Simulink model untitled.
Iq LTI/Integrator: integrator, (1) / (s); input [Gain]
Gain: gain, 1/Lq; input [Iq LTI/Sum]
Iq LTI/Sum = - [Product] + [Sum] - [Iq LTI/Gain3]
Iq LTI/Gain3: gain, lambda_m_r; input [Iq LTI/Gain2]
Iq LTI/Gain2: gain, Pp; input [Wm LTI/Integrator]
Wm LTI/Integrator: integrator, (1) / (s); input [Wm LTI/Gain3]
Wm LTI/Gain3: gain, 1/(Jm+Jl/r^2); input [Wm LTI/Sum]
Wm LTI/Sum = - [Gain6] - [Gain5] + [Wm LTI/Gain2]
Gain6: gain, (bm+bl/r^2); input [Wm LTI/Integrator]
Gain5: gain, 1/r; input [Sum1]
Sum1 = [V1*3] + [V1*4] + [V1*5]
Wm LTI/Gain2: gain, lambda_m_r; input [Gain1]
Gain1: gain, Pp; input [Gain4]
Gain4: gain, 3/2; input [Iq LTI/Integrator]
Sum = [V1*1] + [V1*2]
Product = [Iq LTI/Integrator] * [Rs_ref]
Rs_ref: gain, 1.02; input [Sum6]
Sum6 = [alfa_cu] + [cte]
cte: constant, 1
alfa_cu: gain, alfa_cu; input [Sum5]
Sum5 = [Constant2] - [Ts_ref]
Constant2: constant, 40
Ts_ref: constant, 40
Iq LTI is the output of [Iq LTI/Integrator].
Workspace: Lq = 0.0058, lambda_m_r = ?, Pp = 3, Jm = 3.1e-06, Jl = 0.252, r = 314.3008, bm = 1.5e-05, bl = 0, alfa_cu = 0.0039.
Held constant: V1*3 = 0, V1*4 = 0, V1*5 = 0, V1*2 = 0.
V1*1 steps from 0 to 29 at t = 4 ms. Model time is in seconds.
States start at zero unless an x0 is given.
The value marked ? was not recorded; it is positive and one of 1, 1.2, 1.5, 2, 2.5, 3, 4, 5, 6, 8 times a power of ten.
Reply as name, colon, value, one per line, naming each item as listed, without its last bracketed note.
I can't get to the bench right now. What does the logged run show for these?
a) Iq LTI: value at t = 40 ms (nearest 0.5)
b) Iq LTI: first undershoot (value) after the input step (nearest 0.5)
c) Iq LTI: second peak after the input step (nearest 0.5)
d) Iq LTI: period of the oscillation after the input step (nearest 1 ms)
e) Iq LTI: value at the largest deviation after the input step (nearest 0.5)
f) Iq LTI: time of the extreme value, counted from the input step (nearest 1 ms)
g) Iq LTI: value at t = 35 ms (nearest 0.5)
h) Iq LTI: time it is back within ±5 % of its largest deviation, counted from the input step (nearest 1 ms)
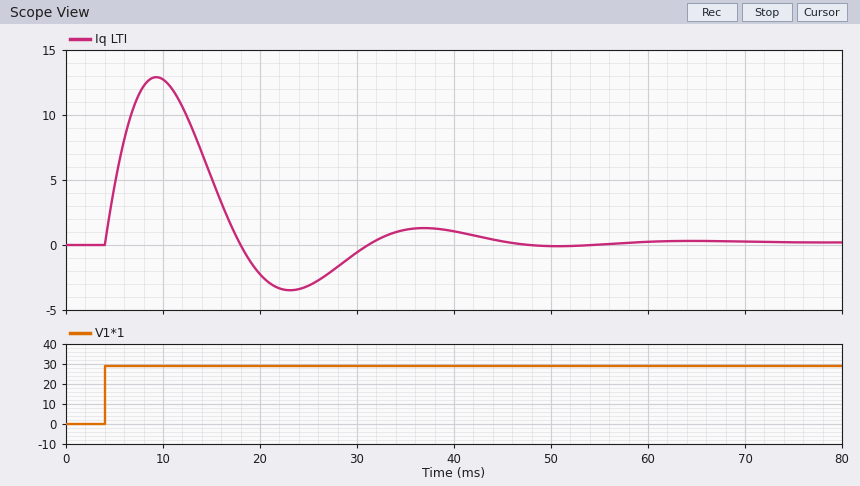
Iq LTI: value at t = 40 ms: 1.0
Iq LTI: first undershoot (value) after the input step: -3.5
Iq LTI: second peak after the input step: 1.5
Iq LTI: period of the oscillation after the input step: 28 ms
Iq LTI: value at the largest deviation after the input step: 13.0
Iq LTI: time of the extreme value, counted from the input step: 5 ms
Iq LTI: value at t = 35 ms: 1.0
Iq LTI: time it is back within ±5 % of its largest deviation, counted from the input step: 37 ms
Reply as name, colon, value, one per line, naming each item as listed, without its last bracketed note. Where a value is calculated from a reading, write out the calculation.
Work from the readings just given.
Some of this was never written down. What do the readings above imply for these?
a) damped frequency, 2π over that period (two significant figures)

damped frequency, 2π over that period: 2π / 28 = 0.22 rad/ms
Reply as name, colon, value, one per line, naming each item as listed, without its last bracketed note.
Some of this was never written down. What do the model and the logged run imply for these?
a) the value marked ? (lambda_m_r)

the value marked ?: 0.012
